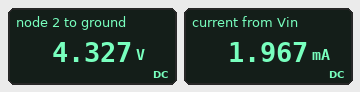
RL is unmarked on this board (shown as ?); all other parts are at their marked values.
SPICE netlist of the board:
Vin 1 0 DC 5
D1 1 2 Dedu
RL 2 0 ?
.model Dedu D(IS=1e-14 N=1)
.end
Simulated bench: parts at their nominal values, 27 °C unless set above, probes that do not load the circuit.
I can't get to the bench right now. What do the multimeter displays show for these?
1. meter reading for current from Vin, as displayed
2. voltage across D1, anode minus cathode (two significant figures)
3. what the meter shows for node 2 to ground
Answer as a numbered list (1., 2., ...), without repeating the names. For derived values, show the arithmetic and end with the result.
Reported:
1. 1.967 mA
2. 5 V - 4.327 V = 670 mV
3. 4.327 V
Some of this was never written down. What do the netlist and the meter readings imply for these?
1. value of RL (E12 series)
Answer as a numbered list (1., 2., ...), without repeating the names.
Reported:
1. 2.2 kΩ
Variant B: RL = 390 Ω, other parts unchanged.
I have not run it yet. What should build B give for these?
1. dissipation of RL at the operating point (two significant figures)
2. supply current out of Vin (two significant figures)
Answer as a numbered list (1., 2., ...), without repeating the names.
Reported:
1. 47 mW
2. 11 mA
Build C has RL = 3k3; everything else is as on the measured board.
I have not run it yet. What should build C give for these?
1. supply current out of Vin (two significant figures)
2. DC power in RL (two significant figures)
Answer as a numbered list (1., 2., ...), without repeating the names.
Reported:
1. 1.3 mA
2. 5.7 mW
